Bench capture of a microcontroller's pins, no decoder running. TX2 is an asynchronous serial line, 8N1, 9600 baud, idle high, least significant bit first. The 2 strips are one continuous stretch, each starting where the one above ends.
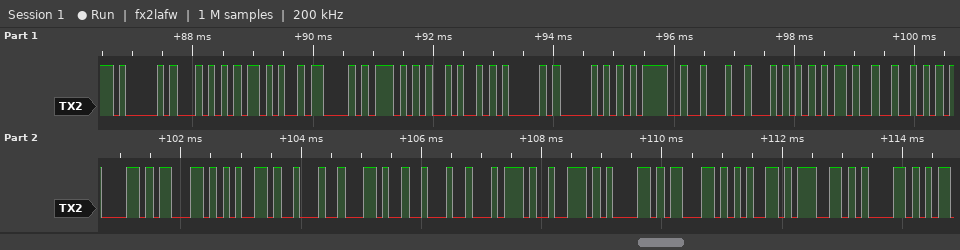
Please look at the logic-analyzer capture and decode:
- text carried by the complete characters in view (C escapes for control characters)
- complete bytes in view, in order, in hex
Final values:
"AT+CWJAP=\"T-Race\",\"tracega"
41 54 2B 43 57 4A 41 50 3D 22 54 2D 52 61 63 65 22 2C 22 74 72 61 63 65 67 61
